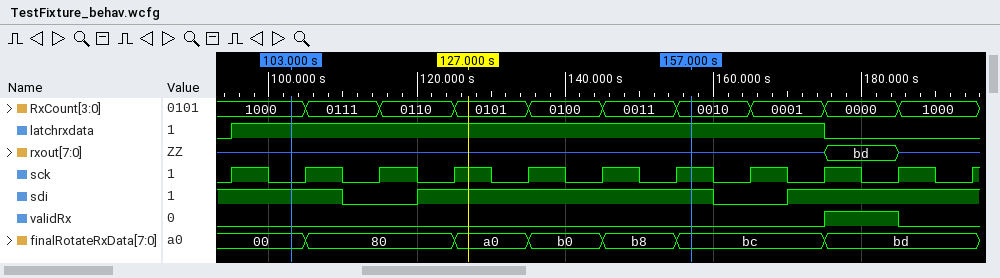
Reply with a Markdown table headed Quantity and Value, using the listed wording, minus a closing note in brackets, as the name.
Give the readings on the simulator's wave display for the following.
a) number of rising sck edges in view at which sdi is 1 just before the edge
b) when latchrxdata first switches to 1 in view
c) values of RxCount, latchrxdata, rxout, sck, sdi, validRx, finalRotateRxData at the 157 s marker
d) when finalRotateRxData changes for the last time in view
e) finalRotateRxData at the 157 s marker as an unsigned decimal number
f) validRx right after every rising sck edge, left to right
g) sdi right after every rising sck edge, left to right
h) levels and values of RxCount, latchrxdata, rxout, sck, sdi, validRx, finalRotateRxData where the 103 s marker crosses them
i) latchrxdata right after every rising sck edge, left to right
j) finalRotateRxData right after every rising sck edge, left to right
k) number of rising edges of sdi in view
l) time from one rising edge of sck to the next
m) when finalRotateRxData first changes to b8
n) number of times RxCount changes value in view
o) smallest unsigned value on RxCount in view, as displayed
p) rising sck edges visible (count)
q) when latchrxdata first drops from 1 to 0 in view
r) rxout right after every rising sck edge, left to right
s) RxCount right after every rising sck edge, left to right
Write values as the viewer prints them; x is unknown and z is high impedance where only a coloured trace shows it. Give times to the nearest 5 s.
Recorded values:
| Quantity | Value |
|---|---|
| number of rising sck edges in view at which sdi is 1 just before the edge | 9 |
| when latchrxdata first switches to 1 in view | 95 s |
| values of RxCount, latchrxdata, rxout, sck, sdi, validRx, finalRotateRxData at the 157 s marker | RxCount=0010, latchrxdata=1, rxout=z, sck=1, sdi=1, validRx=0, finalRotateRxData=bc |
| when finalRotateRxData changes for the last time in view | 175 s |
| finalRotateRxData at the 157 s marker as an unsigned decimal number | 188 |
| validRx right after every rising sck edge, left to right | 0 0 0 0 0 0 0 0 1 0 0 |
| sdi right after every rising sck edge, left to right | 1 1 0 1 1 1 1 0 1 1 1 |
| levels and values of RxCount, latchrxdata, rxout, sck, sdi, validRx, finalRotateRxData where the 103 s marker crosses them | RxCount=1000, latchrxdata=1, rxout=z, sck=0, sdi=1, validRx=0, finalRotateRxData=00 |
| latchrxdata right after every rising sck edge, left to right | 1 1 1 1 1 1 1 1 0 0 0 |
| finalRotateRxData right after every rising sck edge, left to right | 00, 80, 80, a0, b0, b8, bc, bc, bd, bd, bd |
| number of rising edges of sdi in view | 2 |
| time from one rising edge of sck to the next | 10 s |
| when finalRotateRxData first changes to b8 | 145 s |
| number of times RxCount changes value in view | 9 |
| smallest unsigned value on RxCount in view, as displayed | 0000 |
| rising sck edges visible | 11 |
| when latchrxdata first drops from 1 to 0 in view | 175 s |
| rxout right after every rising sck edge, left to right | z, z, z, z, z, z, z, z, bd, z, z |
| RxCount right after every rising sck edge, left to right | 1000, 0111, 0110, 0101, 0100, 0011, 0010, 0001, 0000, 1000, 1000 |
